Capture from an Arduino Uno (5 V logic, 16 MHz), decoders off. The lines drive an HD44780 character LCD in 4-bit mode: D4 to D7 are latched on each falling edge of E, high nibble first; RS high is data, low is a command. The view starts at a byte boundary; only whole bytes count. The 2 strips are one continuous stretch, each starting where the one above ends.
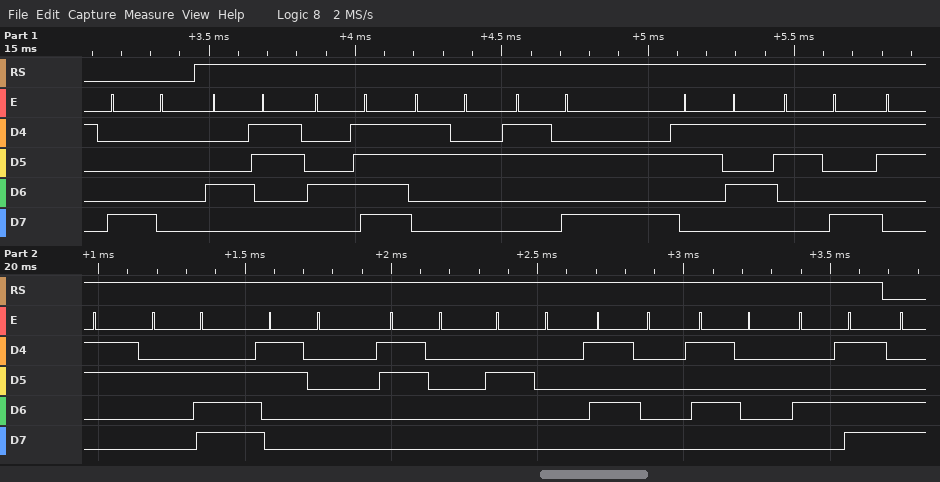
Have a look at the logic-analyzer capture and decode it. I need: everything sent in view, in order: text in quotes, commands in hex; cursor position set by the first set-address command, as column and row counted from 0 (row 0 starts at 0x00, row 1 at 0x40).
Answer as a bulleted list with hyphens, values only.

- 0x80 "CO2:593.00 PPM"
- column 0, row 0
